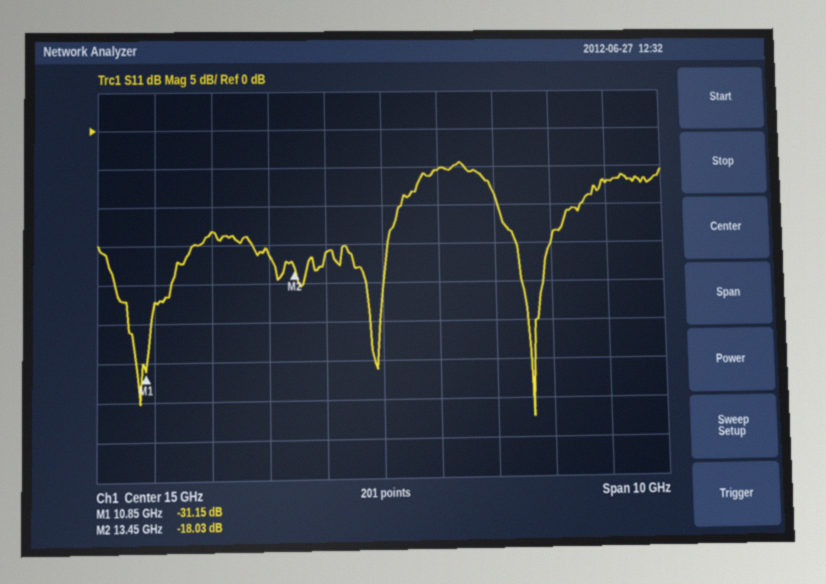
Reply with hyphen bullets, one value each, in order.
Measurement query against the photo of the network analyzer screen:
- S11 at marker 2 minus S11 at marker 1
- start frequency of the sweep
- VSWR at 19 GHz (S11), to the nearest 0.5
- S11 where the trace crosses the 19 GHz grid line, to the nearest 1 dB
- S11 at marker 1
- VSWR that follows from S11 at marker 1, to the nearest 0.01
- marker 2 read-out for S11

- 13.12 dB
- 10 GHz
- 2.5
- -7 dB
- -31.15 dB
- 1.06
- -18.03 dB
